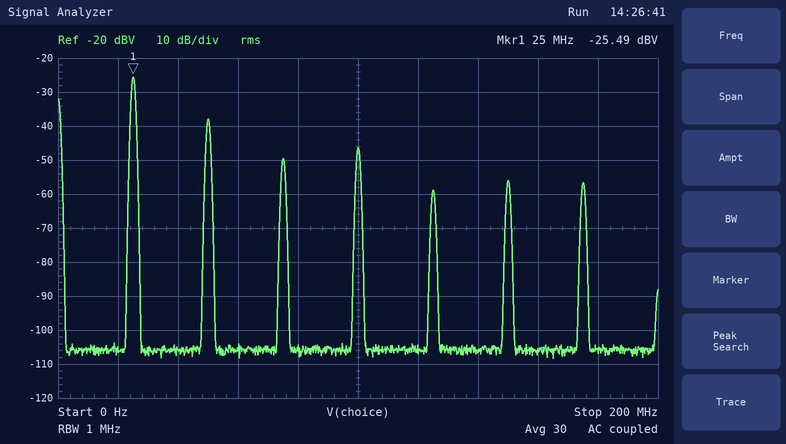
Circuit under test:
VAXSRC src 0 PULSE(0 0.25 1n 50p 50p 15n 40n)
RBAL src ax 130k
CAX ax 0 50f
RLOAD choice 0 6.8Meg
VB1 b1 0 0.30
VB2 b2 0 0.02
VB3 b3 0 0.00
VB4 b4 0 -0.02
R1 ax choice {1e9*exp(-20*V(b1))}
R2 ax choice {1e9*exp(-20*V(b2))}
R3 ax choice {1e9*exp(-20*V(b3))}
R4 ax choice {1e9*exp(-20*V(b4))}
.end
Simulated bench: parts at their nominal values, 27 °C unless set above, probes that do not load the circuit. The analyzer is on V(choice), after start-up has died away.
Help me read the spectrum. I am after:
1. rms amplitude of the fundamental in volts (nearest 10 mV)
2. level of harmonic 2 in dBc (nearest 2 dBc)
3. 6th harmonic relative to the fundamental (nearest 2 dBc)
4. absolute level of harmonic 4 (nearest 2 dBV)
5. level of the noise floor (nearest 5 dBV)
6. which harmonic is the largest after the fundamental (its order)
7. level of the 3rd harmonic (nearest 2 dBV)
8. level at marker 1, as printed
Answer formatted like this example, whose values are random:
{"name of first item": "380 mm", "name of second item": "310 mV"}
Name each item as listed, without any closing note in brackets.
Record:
{"rms amplitude of the fundamental in volts": "50 mV", "level of harmonic 2 in dBc": "-12 dBc", "6th harmonic relative to the fundamental": "-30 dBc", "absolute level of harmonic 4": "-46 dBV", "level of the noise floor": "-105 dBV", "which harmonic is the largest after the fundamental": "2", "level of the 3rd harmonic": "-50 dBV", "level at marker 1, as printed": "-25.49 dBV"}
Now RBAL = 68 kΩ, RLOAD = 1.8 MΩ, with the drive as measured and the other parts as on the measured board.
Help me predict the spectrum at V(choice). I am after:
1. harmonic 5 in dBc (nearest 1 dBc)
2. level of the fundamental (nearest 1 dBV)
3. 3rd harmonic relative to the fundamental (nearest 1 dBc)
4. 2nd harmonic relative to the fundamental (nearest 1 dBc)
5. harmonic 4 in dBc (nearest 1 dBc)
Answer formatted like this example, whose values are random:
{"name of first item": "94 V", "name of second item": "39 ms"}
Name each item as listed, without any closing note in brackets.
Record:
{"harmonic 5 in dBc": "-30 dBc", "level of the fundamental": "-28 dBV", "3rd harmonic relative to the fundamental": "-21 dBc", "2nd harmonic relative to the fundamental": "-11 dBc", "harmonic 4 in dBc": "-18 dBc"}
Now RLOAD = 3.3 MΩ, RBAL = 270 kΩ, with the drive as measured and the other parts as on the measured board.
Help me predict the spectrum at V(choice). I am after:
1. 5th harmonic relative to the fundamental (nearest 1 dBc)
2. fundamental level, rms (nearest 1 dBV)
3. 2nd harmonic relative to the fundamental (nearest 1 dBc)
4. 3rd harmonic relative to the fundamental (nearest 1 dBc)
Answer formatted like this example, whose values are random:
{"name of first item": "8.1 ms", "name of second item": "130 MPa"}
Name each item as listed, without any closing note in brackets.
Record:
{"5th harmonic relative to the fundamental": "-35 dBc", "fundamental level, rms": "-32 dBV", "2nd harmonic relative to the fundamental": "-14 dBc", "3rd harmonic relative to the fundamental": "-26 dBc"}
